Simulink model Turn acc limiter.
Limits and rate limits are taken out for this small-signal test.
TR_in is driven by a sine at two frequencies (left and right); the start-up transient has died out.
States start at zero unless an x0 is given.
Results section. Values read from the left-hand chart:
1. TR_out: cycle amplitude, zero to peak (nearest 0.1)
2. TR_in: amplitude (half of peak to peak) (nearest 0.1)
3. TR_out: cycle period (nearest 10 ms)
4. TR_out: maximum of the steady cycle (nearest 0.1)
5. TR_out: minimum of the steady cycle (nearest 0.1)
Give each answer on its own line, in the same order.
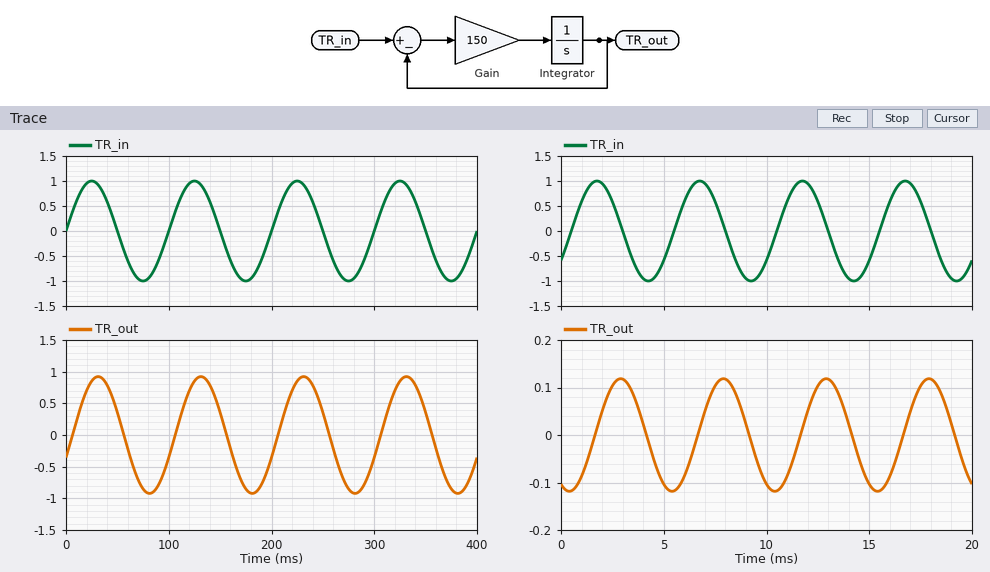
0.9
1.0
100 ms
0.9
-0.9
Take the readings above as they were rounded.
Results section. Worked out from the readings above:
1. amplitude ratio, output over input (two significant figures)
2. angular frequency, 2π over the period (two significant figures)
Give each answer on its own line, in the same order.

0.90
0.063 rad/ms
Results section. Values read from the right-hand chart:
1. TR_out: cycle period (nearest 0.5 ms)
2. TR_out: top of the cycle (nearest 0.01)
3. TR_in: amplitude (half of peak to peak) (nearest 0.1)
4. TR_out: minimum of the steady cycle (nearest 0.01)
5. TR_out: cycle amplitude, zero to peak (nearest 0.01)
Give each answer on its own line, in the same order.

5.0 ms
0.12
1.0
-0.12
0.12
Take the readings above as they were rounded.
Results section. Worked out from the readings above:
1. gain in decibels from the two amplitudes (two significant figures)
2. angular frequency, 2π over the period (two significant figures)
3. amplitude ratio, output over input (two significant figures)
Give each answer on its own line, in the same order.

-18 dB
1.3 rad/ms
0.12
